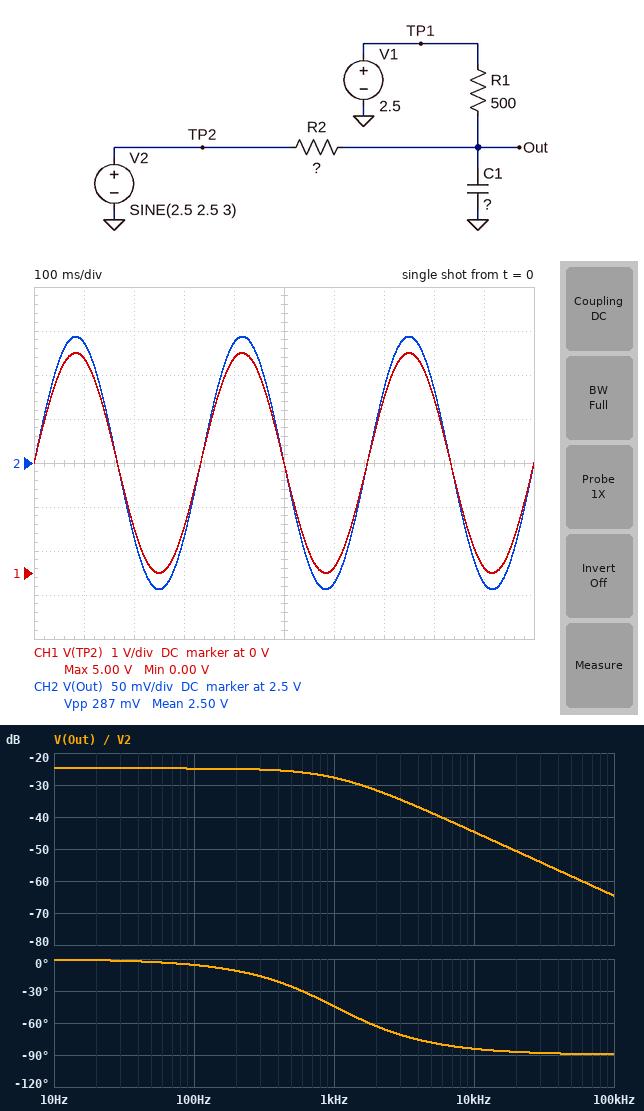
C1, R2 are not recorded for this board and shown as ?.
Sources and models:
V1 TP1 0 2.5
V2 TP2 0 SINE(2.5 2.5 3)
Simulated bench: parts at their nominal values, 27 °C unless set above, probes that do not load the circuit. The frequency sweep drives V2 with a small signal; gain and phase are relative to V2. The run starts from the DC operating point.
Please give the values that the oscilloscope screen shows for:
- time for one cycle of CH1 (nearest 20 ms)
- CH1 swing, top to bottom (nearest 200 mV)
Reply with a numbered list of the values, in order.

1. 340 ms
2. 5.0 V
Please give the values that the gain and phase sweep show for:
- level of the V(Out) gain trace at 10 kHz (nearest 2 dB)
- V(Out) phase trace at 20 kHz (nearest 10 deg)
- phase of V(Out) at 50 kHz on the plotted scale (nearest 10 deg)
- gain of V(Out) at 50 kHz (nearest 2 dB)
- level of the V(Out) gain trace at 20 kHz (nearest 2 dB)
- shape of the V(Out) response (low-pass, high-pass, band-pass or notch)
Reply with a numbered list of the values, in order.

1. -44 dB
2. -90 deg
3. -90 deg
4. -58 dB
5. -50 dB
6. low-pass
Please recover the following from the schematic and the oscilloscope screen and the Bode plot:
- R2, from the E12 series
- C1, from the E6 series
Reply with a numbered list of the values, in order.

1. 8.2 kΩ
2. 330 nF
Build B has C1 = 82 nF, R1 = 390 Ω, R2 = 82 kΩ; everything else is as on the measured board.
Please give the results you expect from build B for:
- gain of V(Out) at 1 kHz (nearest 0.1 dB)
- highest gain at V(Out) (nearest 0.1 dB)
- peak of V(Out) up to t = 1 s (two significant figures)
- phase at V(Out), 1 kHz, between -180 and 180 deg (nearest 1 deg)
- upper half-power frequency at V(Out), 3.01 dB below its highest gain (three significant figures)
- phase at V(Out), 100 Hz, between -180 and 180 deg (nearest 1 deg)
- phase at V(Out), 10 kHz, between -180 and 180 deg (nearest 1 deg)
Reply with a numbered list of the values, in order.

1. -46.7 dB
2. -46.5 dB
3. 2.5 V
4. -11 deg
5. 5.00 kHz
6. -1 deg
7. -63 deg
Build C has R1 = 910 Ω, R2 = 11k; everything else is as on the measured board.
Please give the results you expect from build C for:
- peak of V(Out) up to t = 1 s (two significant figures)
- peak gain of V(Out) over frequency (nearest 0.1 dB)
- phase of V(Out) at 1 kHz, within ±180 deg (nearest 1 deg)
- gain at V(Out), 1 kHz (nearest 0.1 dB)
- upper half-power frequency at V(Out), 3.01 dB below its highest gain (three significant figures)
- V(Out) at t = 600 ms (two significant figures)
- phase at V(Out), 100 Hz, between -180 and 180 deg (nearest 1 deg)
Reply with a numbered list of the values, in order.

1. 2.7 V
2. -22.3 dB
3. -60 deg
4. -28.4 dB
5. 574 Hz
6. 2.3 V
7. -10 deg
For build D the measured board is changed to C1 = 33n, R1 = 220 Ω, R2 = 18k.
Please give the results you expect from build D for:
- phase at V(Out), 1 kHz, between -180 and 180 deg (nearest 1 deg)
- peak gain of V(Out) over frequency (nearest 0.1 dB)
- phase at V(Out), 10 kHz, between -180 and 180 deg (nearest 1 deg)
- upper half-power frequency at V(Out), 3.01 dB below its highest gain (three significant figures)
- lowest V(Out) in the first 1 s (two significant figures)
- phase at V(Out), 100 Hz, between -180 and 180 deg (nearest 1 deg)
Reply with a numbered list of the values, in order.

1. -3 deg
2. -38.4 dB
3. -24 deg
4. 22.2 kHz
5. 2.5 V
6. 0 deg
